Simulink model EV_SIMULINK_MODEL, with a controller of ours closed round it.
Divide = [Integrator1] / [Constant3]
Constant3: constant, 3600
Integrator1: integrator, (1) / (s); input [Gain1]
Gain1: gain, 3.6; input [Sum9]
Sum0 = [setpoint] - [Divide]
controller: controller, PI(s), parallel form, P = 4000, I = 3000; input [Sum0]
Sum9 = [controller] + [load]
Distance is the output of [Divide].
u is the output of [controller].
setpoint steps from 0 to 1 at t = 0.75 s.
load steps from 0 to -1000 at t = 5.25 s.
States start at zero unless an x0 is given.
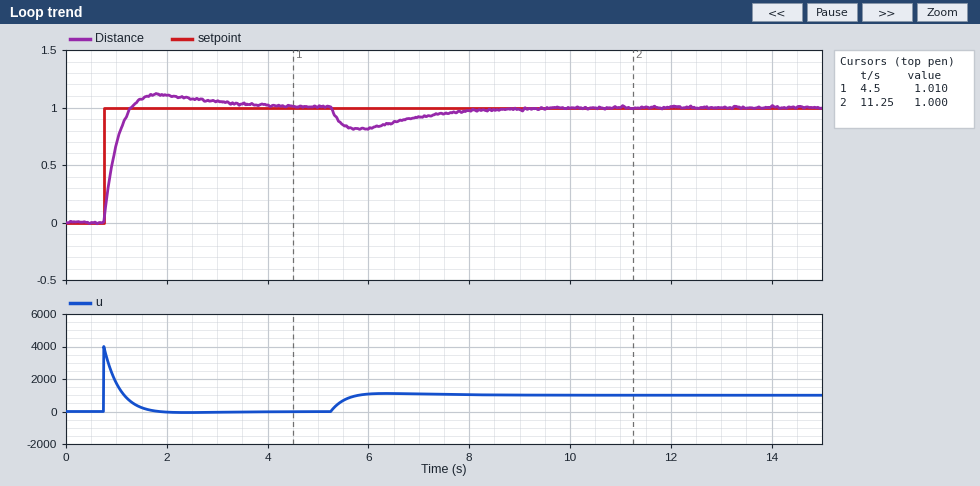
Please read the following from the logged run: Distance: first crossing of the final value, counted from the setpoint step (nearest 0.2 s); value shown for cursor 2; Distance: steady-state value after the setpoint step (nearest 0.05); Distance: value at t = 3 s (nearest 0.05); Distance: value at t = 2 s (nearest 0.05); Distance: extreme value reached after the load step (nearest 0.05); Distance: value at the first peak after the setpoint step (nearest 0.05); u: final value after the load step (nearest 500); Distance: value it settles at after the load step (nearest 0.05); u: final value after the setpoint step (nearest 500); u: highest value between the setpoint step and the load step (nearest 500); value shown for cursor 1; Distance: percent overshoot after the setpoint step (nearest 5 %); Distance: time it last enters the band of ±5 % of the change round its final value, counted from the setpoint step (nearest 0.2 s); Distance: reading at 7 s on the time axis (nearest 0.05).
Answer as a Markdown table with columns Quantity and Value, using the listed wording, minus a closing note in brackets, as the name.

| Quantity | Value |
|---|---|
| Distance: first crossing of the final value, counted from the setpoint step | 0.6 s |
| value shown for cursor 2 | 1.000 |
| Distance: steady-state value after the setpoint step | 1.00 |
| Distance: value at t = 3 s | 1.05 |
| Distance: value at t = 2 s | 1.10 |
| Distance: extreme value reached after the load step | 0.80 |
| Distance: value at the first peak after the setpoint step | 1.10 |
| u: final value after the load step | 1000 |
| Distance: value it settles at after the load step | 1.00 |
| u: final value after the setpoint step | 0 |
| u: highest value between the setpoint step and the load step | 4000 |
| value shown for cursor 1 | 1.010 |
| Distance: percent overshoot after the setpoint step | 10 % |
| Distance: time it last enters the band of ±5 % of the change round its final value, counted from the setpoint step | 2.2 s |
| Distance: reading at 7 s on the time axis | 0.90 |
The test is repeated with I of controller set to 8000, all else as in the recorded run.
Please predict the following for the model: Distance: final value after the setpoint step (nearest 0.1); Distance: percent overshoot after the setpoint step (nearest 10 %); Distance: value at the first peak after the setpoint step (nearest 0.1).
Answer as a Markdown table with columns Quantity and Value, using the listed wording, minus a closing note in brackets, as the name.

| Quantity | Value |
|---|---|
| Distance: final value after the setpoint step | 1.0 |
| Distance: percent overshoot after the setpoint step | 20 % |
| Distance: value at the first peak after the setpoint step | 1.2 |
